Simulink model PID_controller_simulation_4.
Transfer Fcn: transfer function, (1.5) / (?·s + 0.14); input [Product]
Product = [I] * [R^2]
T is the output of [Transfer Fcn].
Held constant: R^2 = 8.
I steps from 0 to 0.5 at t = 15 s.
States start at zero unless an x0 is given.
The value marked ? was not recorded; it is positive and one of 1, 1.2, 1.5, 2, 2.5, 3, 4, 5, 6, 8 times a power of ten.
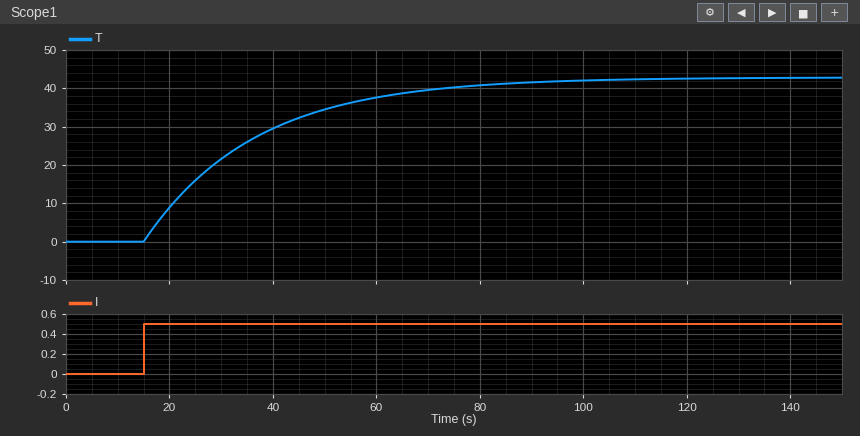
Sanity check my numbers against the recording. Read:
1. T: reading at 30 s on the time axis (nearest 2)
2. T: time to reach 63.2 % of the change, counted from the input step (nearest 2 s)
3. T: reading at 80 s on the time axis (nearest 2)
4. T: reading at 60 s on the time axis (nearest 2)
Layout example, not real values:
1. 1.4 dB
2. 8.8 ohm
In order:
1. 22
2. 22 s
3. 40
4. 38
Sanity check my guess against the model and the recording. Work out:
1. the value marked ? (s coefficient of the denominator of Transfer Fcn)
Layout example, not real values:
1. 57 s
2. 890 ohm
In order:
1. 3
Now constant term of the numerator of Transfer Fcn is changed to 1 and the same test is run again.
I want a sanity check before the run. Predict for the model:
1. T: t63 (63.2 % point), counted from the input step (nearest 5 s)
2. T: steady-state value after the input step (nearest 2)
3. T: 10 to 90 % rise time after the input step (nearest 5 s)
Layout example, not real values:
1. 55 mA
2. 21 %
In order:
1. 20 s
2. 28
3. 45 s
